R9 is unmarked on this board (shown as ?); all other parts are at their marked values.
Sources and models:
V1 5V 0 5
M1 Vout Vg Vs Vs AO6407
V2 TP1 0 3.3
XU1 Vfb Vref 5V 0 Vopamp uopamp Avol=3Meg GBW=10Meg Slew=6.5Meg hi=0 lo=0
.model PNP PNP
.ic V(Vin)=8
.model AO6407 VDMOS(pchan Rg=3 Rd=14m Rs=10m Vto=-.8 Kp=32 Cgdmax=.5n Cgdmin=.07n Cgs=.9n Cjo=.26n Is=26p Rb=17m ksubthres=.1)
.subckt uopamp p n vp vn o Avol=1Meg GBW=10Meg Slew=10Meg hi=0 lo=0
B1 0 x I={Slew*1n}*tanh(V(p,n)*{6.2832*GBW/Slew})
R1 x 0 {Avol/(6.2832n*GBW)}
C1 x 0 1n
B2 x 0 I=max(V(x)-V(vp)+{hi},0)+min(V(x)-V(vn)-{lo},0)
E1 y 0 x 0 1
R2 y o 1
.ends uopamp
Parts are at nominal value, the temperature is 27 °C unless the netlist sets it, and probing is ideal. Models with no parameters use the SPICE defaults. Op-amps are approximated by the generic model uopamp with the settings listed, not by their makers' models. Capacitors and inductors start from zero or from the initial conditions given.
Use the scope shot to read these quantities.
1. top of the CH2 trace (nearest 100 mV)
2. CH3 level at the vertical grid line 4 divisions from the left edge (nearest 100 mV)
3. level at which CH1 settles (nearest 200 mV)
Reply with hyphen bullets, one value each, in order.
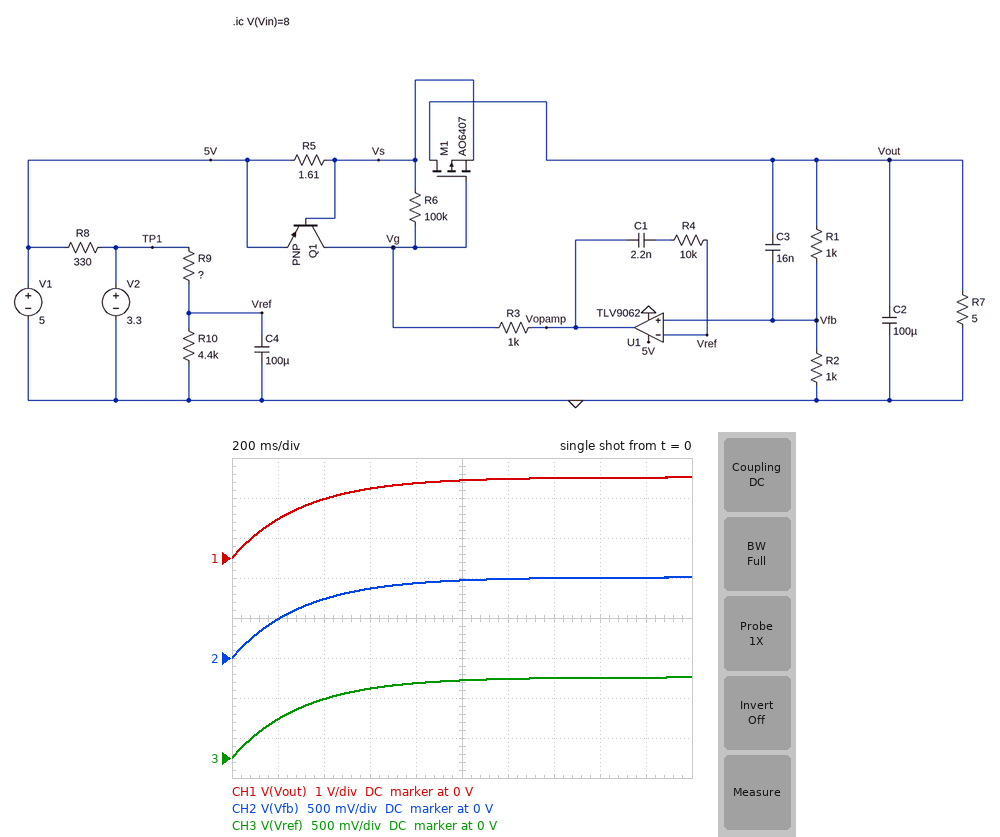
- 1.0 V
- 900 mV
- 2.0 V
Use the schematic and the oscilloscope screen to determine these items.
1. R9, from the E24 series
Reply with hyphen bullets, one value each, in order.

- 10 kΩ
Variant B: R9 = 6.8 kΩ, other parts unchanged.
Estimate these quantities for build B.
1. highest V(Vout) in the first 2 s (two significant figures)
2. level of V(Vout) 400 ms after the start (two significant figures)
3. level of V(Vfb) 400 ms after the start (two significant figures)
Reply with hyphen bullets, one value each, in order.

- 2.5 V
- 2.0 V
- 1.0 V
